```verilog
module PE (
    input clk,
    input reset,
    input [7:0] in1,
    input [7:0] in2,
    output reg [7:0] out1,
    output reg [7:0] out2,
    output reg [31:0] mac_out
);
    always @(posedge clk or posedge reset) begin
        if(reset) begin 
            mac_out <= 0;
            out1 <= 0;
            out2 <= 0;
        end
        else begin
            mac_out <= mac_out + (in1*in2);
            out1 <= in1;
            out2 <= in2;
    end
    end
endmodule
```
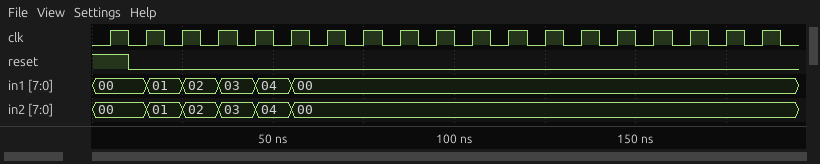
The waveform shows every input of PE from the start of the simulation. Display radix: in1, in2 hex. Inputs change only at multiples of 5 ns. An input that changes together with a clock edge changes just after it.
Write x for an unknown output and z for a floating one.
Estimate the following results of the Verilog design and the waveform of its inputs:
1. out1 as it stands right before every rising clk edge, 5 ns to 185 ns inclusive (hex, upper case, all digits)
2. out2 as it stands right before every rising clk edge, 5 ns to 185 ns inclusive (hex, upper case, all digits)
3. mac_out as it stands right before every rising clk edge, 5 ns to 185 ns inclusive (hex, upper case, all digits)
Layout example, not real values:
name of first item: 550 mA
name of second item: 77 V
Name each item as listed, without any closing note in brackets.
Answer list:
out1 as it stands right before every rising clk edge, 5 ns to 185 ns inclusive: 00, 00, 00, 01, 02, 03, 04, 00, 00, 00, 00, 00, 00, 00, 00, 00, 00, 00, 00
out2 as it stands right before every rising clk edge, 5 ns to 185 ns inclusive: 00, 00, 00, 01, 02, 03, 04, 00, 00, 00, 00, 00, 00, 00, 00, 00, 00, 00, 00
mac_out as it stands right before every rising clk edge, 5 ns to 185 ns inclusive: 00000000, 00000000, 00000000, 00000001, 00000005, 0000000E, 0000001E, 0000001E, 0000001E, 0000001E, 0000001E, 0000001E, 0000001E, 0000001E, 0000001E, 0000001E, 0000001E, 0000001E, 0000001E
